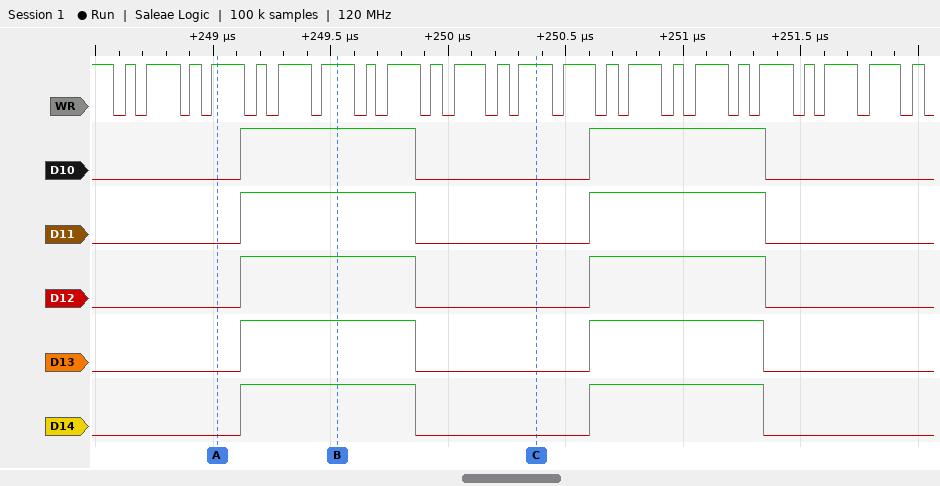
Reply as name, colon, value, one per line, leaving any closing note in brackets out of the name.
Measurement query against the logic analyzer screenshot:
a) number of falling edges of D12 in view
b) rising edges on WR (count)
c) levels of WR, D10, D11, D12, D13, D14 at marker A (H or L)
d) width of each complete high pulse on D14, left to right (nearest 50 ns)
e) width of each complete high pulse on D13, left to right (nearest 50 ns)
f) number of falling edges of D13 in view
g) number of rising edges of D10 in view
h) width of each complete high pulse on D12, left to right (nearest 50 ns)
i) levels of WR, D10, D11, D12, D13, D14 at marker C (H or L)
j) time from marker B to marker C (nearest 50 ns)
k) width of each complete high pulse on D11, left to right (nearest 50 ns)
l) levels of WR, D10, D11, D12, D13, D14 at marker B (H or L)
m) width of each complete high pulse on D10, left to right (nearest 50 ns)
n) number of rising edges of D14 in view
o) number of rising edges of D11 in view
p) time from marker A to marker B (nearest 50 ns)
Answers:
number of falling edges of D12 in view: 2
rising edges on WR: 24
levels of WR, D10, D11, D12, D13, D14 at marker A: WR=H, D10=L, D11=L, D12=L, D13=L, D14=L
width of each complete high pulse on D14, left to right: 750 ns, 750 ns
width of each complete high pulse on D13, left to right: 750 ns, 750 ns
number of falling edges of D13 in view: 2
number of rising edges of D10 in view: 2
width of each complete high pulse on D12, left to right: 750 ns, 750 ns
levels of WR, D10, D11, D12, D13, D14 at marker C: WR=H, D10=L, D11=L, D12=L, D13=L, D14=L
time from marker B to marker C: 850 ns
width of each complete high pulse on D11, left to right: 750 ns, 750 ns
levels of WR, D10, D11, D12, D13, D14 at marker B: WR=H, D10=H, D11=H, D12=H, D13=H, D14=H
width of each complete high pulse on D10, left to right: 750 ns, 750 ns
number of rising edges of D14 in view: 2
number of rising edges of D11 in view: 2
time from marker A to marker B: 500 ns
